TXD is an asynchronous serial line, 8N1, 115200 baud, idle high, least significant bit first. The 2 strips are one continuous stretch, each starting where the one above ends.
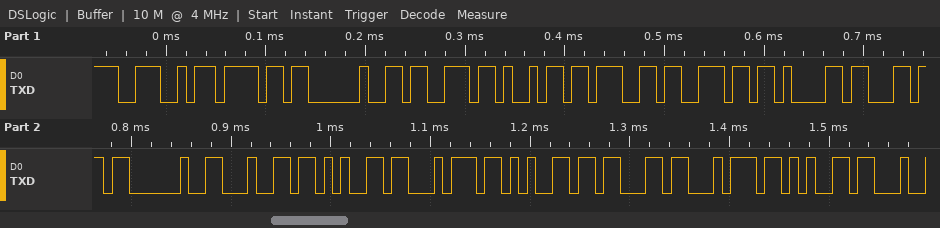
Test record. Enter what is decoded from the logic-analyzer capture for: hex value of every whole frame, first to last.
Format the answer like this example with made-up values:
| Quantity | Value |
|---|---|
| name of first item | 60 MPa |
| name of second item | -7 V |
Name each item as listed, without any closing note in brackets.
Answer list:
| Quantity | Value |
|---|---|
| hex value of every whole frame, first to last | 0x4E 0x6F 0x20 0x73 0x69 0x67 0x6E 0x61 0x6C 0x20 0x64 0x65 0x74 0x65 0x63 0x74 0x65 |
